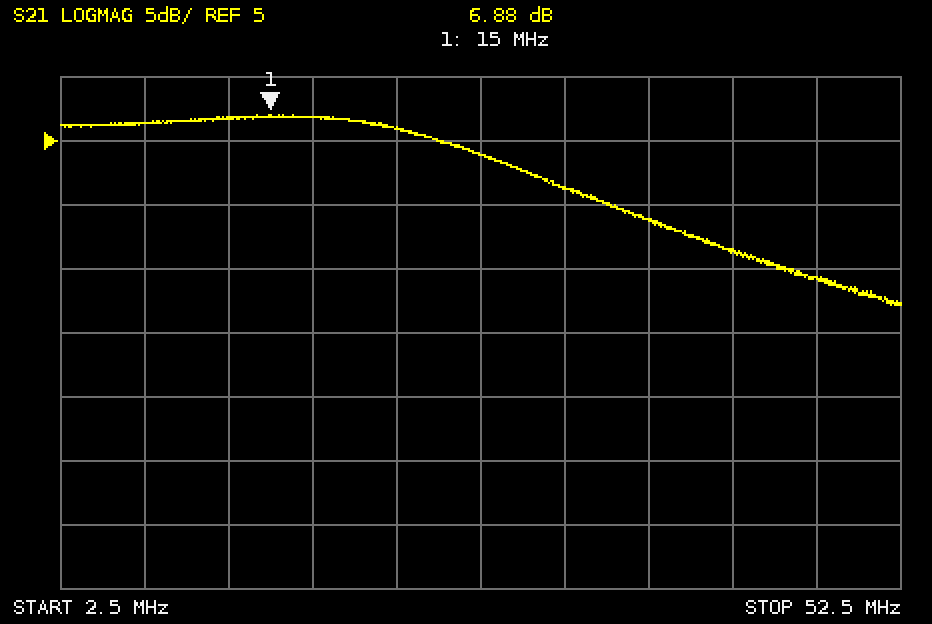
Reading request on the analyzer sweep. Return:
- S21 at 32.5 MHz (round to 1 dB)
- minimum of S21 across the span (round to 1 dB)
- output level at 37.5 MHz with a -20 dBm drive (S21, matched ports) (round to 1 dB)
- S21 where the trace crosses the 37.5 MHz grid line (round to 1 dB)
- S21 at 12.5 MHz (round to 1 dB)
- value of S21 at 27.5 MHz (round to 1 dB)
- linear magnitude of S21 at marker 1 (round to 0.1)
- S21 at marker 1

1 dB
-8 dB
-21 dBm
-1 dB
7 dB
4 dB
2.2
6.88 dB
